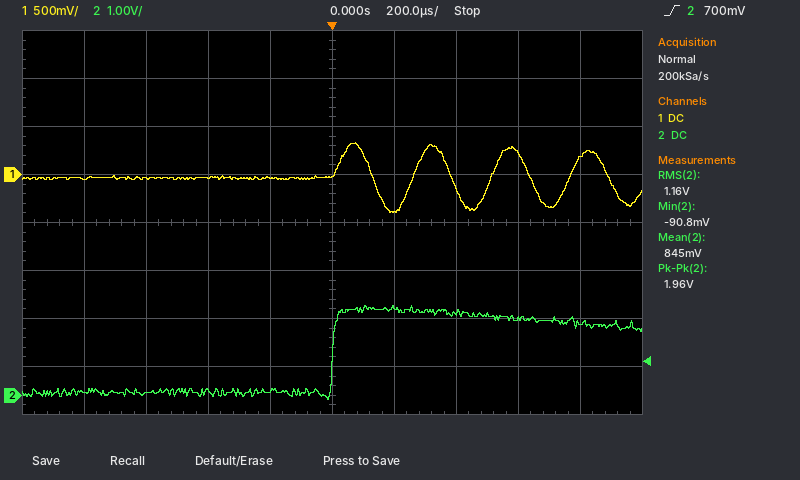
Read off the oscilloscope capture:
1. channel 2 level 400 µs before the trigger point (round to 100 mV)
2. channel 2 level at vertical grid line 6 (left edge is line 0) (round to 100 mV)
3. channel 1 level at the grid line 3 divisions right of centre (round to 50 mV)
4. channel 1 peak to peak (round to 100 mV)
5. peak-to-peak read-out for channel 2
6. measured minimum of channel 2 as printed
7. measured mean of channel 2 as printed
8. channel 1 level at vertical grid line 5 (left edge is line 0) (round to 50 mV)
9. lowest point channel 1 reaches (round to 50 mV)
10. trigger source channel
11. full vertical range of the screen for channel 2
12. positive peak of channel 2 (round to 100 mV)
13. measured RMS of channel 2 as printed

100 mV
1.8 V
200 mV
700 mV
1.96 V
-90.8 mV
845 mV
0 mV
-400 mV
channel 2
8 V
1.9 V
1.16 V
